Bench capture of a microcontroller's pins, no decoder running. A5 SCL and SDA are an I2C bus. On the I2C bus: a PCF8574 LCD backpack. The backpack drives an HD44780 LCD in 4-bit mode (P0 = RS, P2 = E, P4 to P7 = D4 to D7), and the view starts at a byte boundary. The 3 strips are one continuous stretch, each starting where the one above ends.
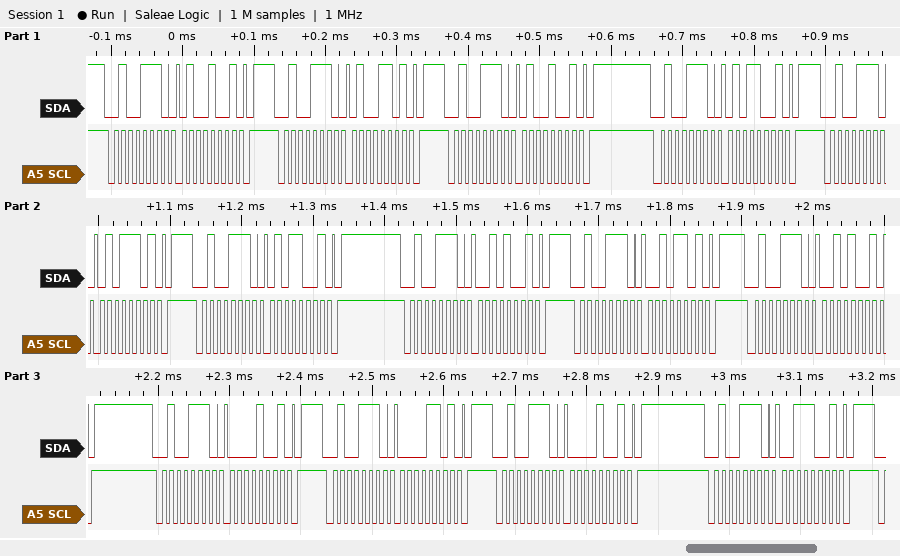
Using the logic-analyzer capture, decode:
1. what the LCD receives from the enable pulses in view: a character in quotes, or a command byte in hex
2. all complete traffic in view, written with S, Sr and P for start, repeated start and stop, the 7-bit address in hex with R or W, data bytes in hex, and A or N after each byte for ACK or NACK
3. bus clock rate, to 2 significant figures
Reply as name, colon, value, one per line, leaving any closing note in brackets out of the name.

what the LCD receives from the enable pulses in view: a character in quotes, or a command byte in hex: 'E' ' '
all complete traffic in view, written with S, Sr and P for start, repeated start and stop, the 7-bit address in hex with R or W, data bytes in hex, and A or N after each byte for ACK or NACK: S 27W A 49 A P S 27W A 4D A P S 27W A 49 A P S 27W A 59 A P S 27W A 5D A P S 27W A 59 A P S 27W A 29 A P S 27W A 2D A P S 27W A 29 A P S 27W A 09 A P S 27W A 0D A P S 27W A 09 A P S 27W A 39 A P
bus clock rate, to 2 significant figures: 100 kHz
